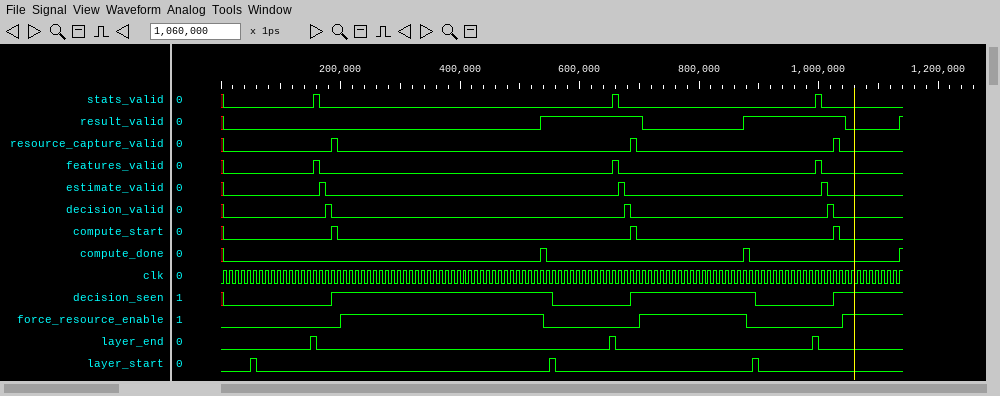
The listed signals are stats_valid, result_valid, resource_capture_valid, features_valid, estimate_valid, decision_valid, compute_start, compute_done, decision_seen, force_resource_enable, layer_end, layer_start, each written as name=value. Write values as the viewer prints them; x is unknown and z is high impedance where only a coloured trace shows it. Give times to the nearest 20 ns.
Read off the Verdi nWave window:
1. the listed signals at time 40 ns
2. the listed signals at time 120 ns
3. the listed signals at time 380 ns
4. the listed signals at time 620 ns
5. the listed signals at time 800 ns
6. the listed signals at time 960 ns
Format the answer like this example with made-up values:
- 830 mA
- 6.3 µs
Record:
- stats_valid=0, result_valid=0, resource_capture_valid=0, features_valid=0, estimate_valid=0, decision_valid=0, compute_start=0, compute_done=0, decision_seen=0, force_resource_enable=0, layer_end=0, layer_start=0
- stats_valid=0, result_valid=0, resource_capture_valid=0, features_valid=0, estimate_valid=0, decision_valid=0, compute_start=0, compute_done=0, decision_seen=0, force_resource_enable=0, layer_end=0, layer_start=0
- stats_valid=0, result_valid=0, resource_capture_valid=0, features_valid=0, estimate_valid=0, decision_valid=0, compute_start=0, compute_done=0, decision_seen=1, force_resource_enable=1, layer_end=0, layer_start=0
- stats_valid=0, result_valid=1, resource_capture_valid=0, features_valid=0, estimate_valid=0, decision_valid=0, compute_start=0, compute_done=0, decision_seen=0, force_resource_enable=0, layer_end=0, layer_start=0
- stats_valid=0, result_valid=0, resource_capture_valid=0, features_valid=0, estimate_valid=0, decision_valid=0, compute_start=0, compute_done=0, decision_seen=1, force_resource_enable=1, layer_end=0, layer_start=0
- stats_valid=0, result_valid=1, resource_capture_valid=0, features_valid=0, estimate_valid=0, decision_valid=0, compute_start=0, compute_done=0, decision_seen=0, force_resource_enable=0, layer_end=0, layer_start=0
